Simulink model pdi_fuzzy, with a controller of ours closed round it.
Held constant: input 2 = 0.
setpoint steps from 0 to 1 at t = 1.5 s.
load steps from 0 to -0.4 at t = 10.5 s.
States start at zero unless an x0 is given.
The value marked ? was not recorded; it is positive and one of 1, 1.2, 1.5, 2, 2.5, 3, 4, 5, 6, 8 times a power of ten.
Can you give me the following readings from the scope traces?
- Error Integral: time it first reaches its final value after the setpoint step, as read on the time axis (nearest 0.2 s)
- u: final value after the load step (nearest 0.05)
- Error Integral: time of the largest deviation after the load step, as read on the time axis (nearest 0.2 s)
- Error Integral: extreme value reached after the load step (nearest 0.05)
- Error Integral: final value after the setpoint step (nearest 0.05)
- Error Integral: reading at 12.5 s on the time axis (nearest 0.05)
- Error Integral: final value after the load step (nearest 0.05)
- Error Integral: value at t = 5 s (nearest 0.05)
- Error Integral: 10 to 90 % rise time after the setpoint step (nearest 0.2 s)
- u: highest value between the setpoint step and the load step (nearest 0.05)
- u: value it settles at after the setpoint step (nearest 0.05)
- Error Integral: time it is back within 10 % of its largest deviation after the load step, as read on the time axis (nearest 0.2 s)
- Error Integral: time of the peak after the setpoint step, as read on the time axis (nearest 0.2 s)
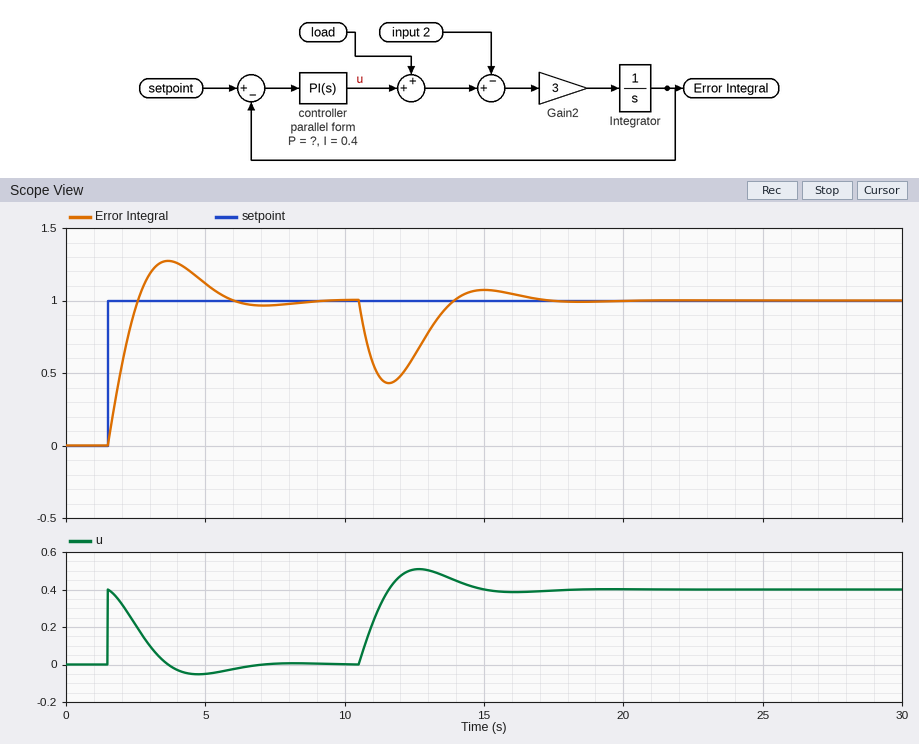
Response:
2.6 s
0.40
11.6 s
0.45
1.00
0.60
1.00
1.10
0.8 s
0.40
0.00
15.8 s
3.6 s
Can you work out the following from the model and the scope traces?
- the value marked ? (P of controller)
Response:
0.4
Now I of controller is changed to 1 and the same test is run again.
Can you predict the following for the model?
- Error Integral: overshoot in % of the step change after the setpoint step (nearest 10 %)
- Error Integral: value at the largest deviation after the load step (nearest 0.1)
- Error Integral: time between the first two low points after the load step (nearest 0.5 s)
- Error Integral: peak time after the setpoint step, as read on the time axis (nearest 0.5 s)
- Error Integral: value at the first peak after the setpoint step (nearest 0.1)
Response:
40 %
0.6
4.0 s
3.0 s
1.4
